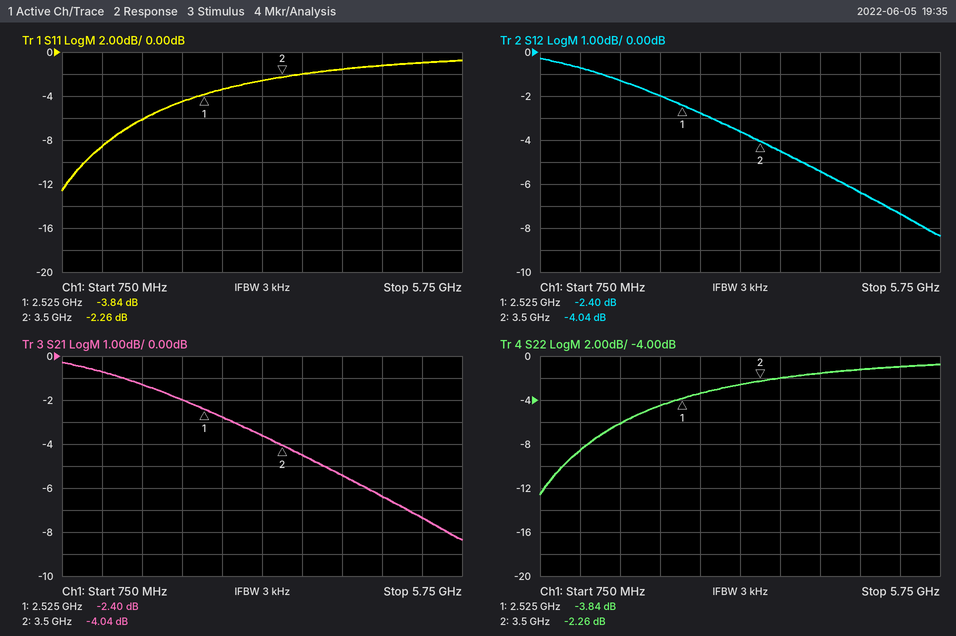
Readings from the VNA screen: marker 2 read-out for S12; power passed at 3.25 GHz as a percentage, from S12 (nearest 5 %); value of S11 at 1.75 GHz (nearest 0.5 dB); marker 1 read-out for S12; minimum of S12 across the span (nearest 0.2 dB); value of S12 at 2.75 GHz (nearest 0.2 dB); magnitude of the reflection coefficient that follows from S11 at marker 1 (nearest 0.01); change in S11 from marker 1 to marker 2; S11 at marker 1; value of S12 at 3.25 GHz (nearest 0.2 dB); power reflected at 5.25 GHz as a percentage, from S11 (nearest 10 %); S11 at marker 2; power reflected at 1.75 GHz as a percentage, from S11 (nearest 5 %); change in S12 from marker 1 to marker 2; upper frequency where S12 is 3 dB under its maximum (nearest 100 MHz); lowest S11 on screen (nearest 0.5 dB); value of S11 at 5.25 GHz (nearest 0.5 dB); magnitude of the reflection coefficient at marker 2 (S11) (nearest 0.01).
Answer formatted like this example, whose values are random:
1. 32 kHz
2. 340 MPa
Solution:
1. -4.04 dB
2. 45 %
3. -6.0 dB
4. -2.40 dB
5. -8.4 dB
6. -2.8 dB
7. 0.64
8. 1.58 dB
9. -3.84 dB
10. -3.6 dB
11. 80 %
12. -2.26 dB
13. 25 %
14. -1.64 dB
15. 3.1 GHz
16. -12.5 dB
17. -1.0 dB
18. 0.77
